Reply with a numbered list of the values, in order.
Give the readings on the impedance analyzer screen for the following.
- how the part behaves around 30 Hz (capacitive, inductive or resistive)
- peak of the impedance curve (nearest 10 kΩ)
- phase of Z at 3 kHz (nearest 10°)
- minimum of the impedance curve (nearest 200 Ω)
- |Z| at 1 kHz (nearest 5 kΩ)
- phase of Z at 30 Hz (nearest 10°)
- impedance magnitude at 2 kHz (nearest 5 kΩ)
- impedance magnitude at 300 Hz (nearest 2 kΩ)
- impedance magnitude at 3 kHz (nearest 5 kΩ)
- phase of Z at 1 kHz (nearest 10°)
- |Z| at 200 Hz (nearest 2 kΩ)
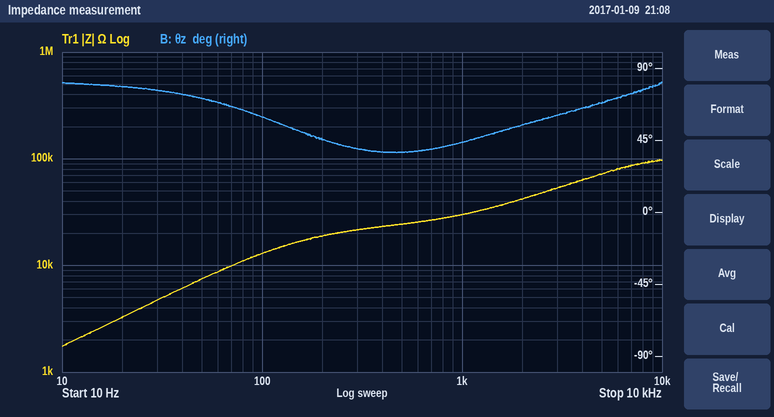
1. inductive
2. 100 kΩ
3. 60°
4. 1.8 kΩ
5. 30 kΩ
6. 80°
7. 40 kΩ
8. 22 kΩ
9. 55 kΩ
10. 40°
11. 18 kΩ
